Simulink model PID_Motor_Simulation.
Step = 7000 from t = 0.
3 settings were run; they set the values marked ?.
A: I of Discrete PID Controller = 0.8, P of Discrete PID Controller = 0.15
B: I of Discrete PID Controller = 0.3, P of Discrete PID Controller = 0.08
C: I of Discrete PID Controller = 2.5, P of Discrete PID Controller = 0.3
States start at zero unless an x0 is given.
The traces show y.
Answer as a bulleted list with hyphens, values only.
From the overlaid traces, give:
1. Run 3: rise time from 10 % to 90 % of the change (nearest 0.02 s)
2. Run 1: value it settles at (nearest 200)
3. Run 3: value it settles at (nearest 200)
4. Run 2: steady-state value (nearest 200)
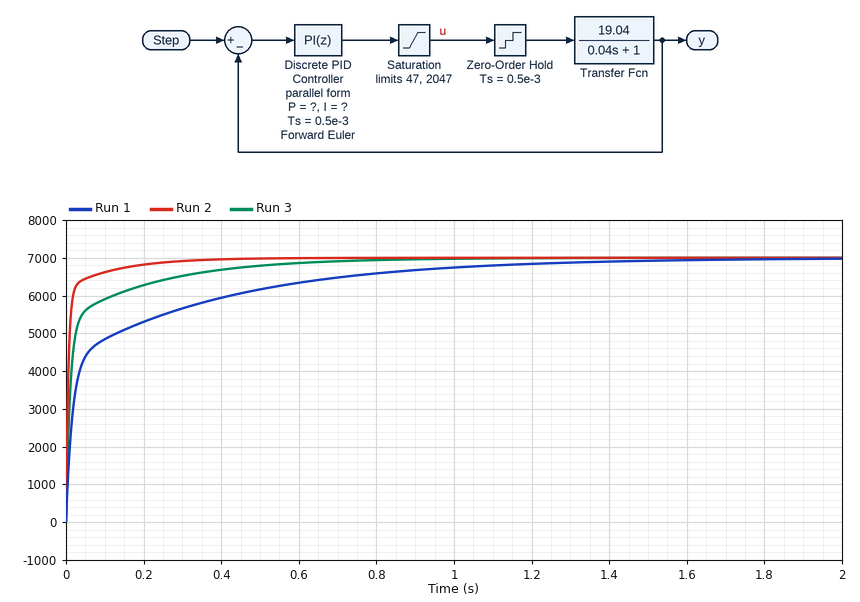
- 0.20 s
- 7000
- 7000
- 7000
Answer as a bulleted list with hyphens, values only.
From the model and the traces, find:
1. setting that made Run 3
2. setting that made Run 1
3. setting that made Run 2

- A
- B
- C
